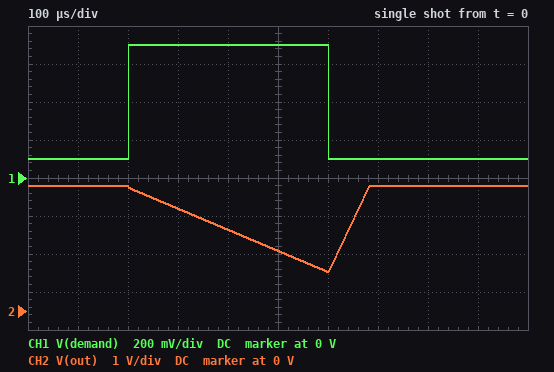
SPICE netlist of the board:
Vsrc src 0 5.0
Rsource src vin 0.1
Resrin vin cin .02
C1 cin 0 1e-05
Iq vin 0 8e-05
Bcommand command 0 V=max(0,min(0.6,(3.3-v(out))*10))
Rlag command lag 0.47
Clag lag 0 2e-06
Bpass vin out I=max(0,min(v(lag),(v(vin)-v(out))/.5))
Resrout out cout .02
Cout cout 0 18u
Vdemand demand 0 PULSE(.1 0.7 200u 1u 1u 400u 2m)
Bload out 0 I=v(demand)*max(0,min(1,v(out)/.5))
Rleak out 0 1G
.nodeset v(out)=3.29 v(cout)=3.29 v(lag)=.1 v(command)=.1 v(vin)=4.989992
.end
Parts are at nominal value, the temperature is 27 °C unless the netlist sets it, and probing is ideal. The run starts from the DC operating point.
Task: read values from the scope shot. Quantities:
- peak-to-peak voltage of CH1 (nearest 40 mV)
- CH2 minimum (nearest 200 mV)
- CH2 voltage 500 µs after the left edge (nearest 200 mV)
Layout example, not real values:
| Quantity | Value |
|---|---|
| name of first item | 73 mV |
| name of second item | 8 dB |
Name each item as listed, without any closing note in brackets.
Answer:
| Quantity | Value |
|---|---|
| peak-to-peak voltage of CH1 | 600 mV |
| CH2 minimum | 1.0 V |
| CH2 voltage 500 µs after the left edge | 1.6 V |
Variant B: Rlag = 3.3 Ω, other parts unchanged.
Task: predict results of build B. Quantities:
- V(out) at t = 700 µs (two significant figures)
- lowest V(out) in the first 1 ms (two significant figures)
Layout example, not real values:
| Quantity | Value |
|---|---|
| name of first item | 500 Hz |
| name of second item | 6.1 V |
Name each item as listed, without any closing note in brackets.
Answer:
| Quantity | Value |
|---|---|
| V(out) at t = 700 µs | 3.4 V |
| lowest V(out) in the first 1 ms | 870 mV |
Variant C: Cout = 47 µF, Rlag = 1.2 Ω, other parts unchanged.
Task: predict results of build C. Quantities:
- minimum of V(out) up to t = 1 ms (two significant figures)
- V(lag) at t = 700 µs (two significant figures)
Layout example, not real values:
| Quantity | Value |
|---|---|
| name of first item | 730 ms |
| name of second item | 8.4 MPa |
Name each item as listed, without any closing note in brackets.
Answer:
| Quantity | Value |
|---|---|
| minimum of V(out) up to t = 1 ms | 2.4 V |
| V(lag) at t = 700 µs | 96 mV |
